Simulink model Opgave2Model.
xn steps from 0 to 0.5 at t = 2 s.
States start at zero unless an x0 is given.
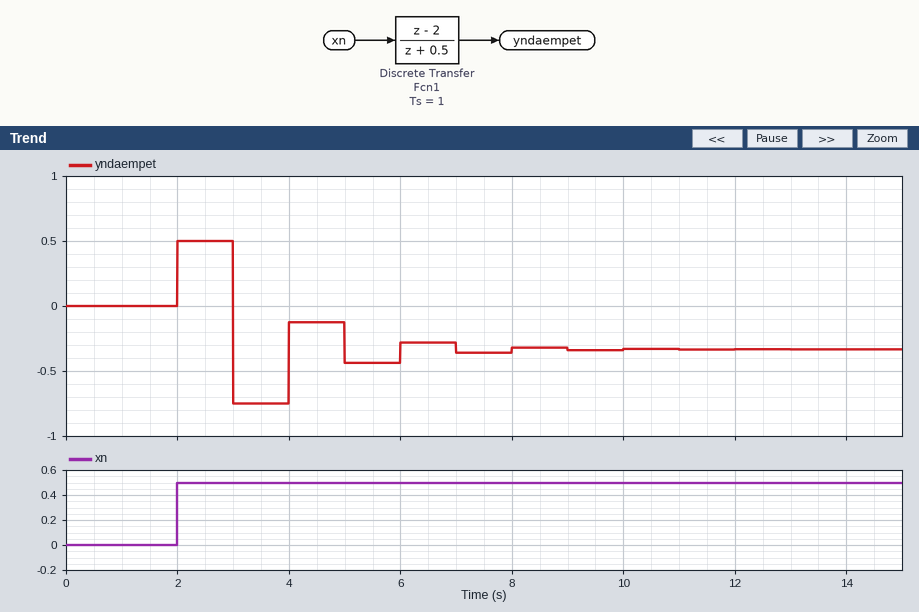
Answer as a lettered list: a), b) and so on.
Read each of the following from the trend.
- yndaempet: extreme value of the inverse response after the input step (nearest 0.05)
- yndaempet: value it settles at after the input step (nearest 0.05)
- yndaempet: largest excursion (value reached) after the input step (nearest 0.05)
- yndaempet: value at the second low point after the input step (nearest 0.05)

a) 0.50
b) -0.35
c) -0.75
d) -0.45
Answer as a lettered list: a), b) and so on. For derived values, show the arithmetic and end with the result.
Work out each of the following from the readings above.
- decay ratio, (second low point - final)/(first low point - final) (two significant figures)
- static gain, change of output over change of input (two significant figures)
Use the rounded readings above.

a) (-0.45 - (-0.35)) / (-0.75 - (-0.35)) = 0.25
b) (-0.35 - 0) / (0.5 - 0) = -0.70
